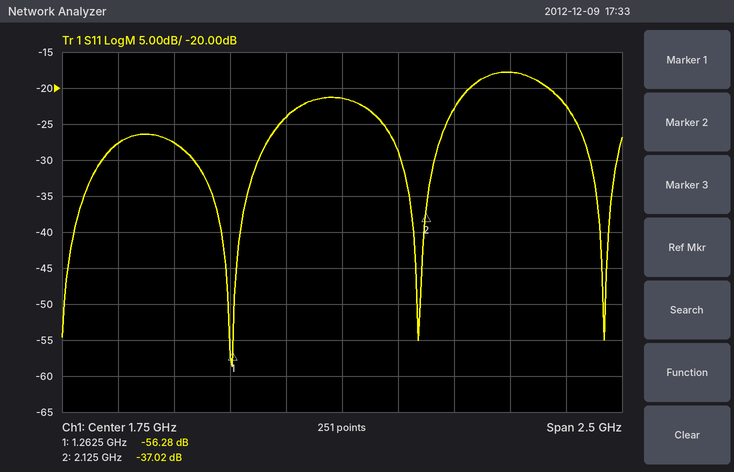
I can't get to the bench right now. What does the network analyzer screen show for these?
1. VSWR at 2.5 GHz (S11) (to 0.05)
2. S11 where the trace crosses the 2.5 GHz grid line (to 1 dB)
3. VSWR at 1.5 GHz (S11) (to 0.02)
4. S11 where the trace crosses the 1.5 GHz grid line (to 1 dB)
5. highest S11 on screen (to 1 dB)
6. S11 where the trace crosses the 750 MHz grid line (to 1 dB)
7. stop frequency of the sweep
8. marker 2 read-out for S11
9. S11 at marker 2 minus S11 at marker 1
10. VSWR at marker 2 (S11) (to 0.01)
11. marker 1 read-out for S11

1.30
-18 dB
1.14
-24 dB
-18 dB
-28 dB
3 GHz
-37.02 dB
19.26 dB
1.03
-56.28 dB
